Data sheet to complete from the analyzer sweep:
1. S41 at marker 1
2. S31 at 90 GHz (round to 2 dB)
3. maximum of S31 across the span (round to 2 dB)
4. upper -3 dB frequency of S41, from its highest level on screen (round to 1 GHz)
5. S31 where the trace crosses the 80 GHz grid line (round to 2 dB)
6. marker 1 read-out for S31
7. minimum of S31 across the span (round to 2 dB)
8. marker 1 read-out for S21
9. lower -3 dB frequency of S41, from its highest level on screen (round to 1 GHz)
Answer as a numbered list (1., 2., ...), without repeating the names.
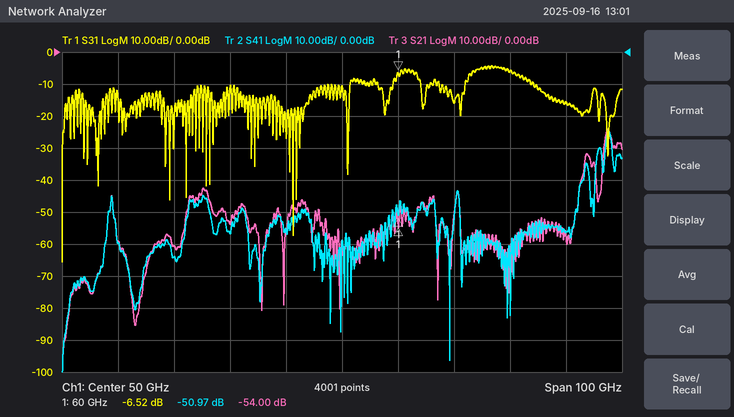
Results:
1. -50.97 dB
2. -16 dB
3. -4 dB
4. 98 GHz
5. -6 dB
6. -6.52 dB
7. -66 dB
8. -54.00 dB
9. 97 GHz
